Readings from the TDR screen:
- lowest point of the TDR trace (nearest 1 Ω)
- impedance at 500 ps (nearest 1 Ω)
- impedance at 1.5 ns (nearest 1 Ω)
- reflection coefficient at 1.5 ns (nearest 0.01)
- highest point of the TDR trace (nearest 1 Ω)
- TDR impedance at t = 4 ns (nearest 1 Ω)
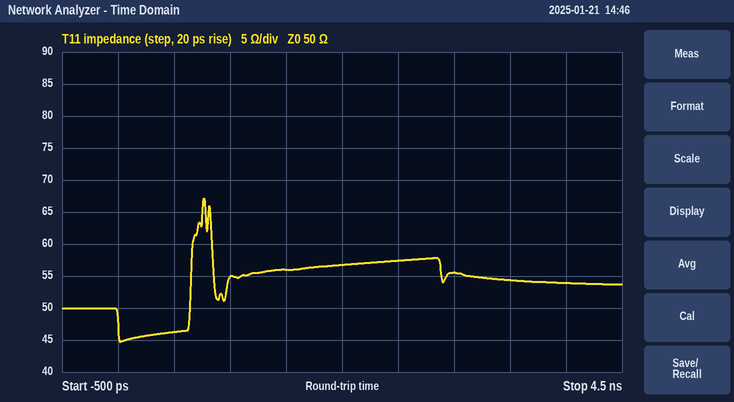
45 Ω
46 Ω
56 Ω
+0.06
67 Ω
54 Ω
